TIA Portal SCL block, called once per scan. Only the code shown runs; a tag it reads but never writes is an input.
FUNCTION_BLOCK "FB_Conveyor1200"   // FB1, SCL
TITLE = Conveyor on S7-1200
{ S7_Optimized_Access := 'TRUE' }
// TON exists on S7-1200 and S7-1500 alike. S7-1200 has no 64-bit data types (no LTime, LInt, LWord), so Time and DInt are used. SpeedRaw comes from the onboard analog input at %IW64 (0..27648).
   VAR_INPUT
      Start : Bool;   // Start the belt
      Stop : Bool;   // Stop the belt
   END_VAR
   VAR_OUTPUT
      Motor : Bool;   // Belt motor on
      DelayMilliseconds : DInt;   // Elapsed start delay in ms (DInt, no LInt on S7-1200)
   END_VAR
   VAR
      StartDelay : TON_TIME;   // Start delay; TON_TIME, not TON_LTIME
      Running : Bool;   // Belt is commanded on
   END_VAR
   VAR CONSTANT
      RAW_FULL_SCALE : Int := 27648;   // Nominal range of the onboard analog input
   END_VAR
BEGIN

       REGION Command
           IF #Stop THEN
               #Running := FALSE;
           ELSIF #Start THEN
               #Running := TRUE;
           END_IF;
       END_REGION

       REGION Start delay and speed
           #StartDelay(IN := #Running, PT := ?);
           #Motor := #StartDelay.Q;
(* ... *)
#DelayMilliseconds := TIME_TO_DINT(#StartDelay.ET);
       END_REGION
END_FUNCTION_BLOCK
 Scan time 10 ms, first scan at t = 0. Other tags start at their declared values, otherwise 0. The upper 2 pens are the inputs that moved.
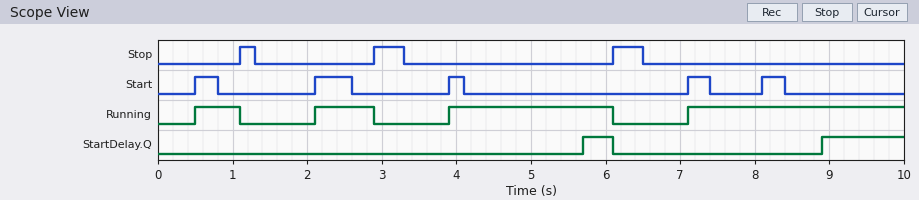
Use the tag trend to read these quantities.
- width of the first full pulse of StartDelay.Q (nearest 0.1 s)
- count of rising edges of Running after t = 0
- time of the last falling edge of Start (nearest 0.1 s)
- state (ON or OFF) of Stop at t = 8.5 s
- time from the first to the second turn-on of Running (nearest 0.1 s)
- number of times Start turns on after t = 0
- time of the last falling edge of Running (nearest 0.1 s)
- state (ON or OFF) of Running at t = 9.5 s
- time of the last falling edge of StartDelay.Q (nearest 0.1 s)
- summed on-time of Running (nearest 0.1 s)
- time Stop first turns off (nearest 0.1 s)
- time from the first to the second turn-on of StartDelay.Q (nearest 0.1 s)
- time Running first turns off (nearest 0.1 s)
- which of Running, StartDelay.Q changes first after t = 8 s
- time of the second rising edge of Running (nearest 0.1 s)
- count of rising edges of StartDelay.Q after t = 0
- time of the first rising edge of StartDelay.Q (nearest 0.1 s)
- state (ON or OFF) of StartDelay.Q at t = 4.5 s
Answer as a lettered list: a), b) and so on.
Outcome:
a) 0.4 s
b) 4
c) 8.4 s
d) OFF
e) 1.6 s
f) 5
g) 6.1 s
h) ON
i) 6.1 s
j) 6.5 s
k) 1.3 s
l) 3.2 s
m) 1.1 s
n) StartDelay.Q
o) 2.1 s
p) 2
q) 5.7 s
r) OFF
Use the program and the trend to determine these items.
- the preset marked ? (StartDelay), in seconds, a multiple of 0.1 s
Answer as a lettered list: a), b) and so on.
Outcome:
a) 1.8 s
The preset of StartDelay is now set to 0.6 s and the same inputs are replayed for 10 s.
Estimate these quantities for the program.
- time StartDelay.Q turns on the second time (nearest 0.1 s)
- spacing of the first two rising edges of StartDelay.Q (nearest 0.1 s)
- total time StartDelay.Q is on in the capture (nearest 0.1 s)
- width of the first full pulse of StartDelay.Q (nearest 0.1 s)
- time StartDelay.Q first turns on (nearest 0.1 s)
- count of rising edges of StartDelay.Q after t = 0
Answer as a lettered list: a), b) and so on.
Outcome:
a) 4.5 s
b) 1.8 s
c) 4.1 s
d) 0.2 s
e) 2.7 s
f) 3
